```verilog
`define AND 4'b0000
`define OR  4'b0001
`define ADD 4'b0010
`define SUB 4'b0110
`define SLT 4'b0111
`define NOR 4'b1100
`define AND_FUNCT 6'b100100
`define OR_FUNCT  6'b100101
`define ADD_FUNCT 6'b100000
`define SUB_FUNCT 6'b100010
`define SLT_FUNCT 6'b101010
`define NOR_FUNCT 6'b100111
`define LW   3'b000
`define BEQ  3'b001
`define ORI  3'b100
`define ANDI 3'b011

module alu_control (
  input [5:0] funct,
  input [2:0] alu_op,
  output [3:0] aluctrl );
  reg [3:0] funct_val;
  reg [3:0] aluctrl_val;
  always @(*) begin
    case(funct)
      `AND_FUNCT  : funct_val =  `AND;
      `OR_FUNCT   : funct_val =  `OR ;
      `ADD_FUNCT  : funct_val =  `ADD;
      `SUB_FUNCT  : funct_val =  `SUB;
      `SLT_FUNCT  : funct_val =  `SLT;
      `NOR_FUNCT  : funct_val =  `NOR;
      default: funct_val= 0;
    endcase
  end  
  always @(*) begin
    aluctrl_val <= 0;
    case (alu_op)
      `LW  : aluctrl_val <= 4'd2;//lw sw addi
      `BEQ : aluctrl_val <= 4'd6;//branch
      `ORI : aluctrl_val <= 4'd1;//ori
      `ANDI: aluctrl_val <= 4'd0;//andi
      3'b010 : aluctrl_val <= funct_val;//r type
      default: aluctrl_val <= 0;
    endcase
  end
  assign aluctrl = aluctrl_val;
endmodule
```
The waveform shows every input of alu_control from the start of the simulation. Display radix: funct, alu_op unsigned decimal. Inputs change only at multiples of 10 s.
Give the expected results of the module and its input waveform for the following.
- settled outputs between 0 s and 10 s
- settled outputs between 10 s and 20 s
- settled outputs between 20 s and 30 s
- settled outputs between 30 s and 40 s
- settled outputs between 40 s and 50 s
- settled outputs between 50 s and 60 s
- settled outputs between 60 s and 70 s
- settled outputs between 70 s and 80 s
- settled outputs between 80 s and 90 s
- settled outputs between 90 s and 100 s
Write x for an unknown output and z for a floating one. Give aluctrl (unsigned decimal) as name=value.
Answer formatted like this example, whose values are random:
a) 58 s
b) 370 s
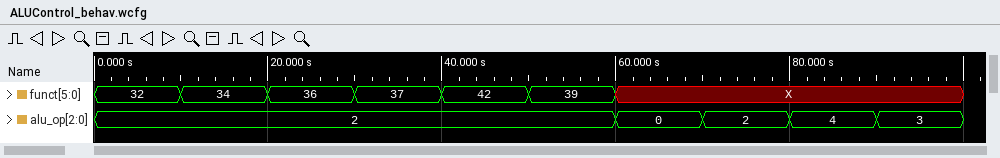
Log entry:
a) aluctrl=2
b) aluctrl=6
c) aluctrl=0
d) aluctrl=1
e) aluctrl=7
f) aluctrl=12
g) aluctrl=2
h) aluctrl=0
i) aluctrl=1
j) aluctrl=0
